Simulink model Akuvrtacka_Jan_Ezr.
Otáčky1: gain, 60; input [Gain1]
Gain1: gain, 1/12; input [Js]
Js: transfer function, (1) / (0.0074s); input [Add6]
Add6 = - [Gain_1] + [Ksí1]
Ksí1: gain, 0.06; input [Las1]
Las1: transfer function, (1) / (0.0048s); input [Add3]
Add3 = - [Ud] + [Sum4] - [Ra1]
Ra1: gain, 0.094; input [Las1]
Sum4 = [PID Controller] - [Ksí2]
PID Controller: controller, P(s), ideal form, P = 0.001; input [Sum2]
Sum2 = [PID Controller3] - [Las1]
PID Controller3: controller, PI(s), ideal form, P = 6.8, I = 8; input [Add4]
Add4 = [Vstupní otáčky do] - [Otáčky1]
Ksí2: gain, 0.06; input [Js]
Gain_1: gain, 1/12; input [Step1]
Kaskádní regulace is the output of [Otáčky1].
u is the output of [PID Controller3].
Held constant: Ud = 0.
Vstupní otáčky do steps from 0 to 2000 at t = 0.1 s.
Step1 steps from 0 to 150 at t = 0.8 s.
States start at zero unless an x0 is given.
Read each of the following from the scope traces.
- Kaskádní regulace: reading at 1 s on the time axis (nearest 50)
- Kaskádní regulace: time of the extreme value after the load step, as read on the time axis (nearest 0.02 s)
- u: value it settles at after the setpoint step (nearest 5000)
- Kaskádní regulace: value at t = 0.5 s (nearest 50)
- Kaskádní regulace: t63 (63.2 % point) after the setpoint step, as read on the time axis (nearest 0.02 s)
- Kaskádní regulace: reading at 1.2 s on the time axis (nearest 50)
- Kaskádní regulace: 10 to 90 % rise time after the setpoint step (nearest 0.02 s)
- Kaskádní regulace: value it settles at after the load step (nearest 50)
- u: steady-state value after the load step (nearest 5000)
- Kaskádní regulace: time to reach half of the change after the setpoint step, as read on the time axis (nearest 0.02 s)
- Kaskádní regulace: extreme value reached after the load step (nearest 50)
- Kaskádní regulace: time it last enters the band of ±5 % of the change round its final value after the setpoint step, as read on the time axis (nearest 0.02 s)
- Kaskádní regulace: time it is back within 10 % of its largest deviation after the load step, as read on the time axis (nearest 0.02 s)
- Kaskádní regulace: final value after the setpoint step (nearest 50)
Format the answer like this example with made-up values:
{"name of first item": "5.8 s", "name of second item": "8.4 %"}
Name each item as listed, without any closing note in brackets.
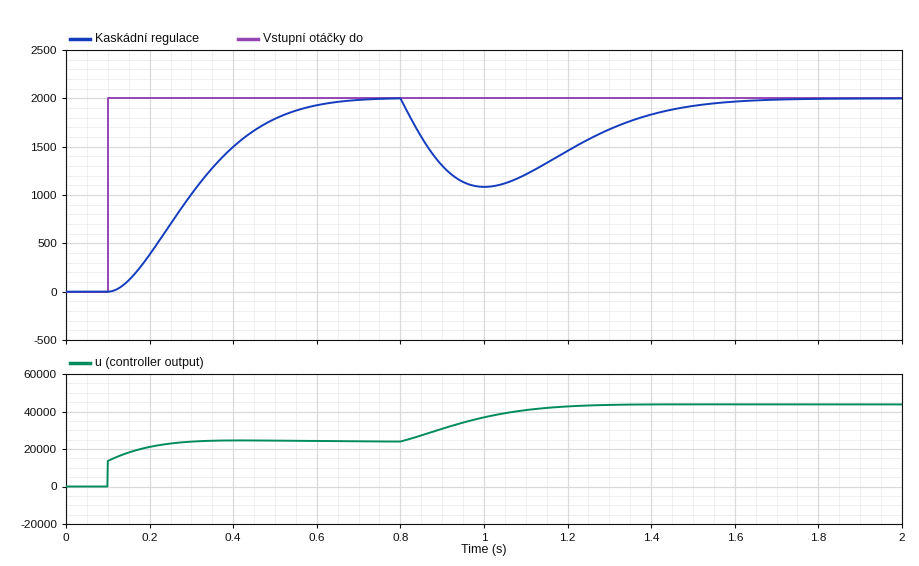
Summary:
{"Kaskádní regulace: reading at 1 s on the time axis": "1100", "Kaskádní regulace: time of the extreme value after the load step, as read on the time axis": "1.00 s", "u: value it settles at after the setpoint step": "25000", "Kaskádní regulace: value at t = 0.5 s": "1800", "Kaskádní regulace: t63 (63.2 % point) after the setpoint step, as read on the time axis": "0.34 s", "Kaskádní regulace: reading at 1.2 s on the time axis": "1450", "Kaskádní regulace: 10 to 90 % rise time after the setpoint step": "0.34 s", "Kaskádní regulace: value it settles at after the load step": "2000", "u: steady-state value after the load step": "45000", "Kaskádní regulace: time to reach half of the change after the setpoint step, as read on the time axis": "0.30 s", "Kaskádní regulace: extreme value reached after the load step": "1100", "Kaskádní regulace: time it last enters the band of ±5 % of the change round its final value after the setpoint step, as read on the time axis": "0.58 s", "Kaskádní regulace: time it is back within 10 % of its largest deviation after the load step, as read on the time axis": "1.48 s", "Kaskádní regulace: final value after the setpoint step": "2000"}
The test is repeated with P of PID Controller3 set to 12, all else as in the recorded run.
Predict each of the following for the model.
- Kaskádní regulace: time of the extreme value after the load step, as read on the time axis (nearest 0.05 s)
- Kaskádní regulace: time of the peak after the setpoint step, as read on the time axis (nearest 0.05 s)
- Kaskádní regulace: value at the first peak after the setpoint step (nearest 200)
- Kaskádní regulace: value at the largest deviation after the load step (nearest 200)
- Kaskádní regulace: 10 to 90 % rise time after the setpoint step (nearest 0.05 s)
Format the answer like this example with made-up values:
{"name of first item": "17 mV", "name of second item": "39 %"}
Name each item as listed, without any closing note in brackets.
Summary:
{"Kaskádní regulace: time of the extreme value after the load step, as read on the time axis": "0.95 s", "Kaskádní regulace: time of the peak after the setpoint step, as read on the time axis": "0.50 s", "Kaskádní regulace: value at the first peak after the setpoint step": "2200", "Kaskádní regulace: value at the largest deviation after the load step": "1200", "Kaskádní regulace: 10 to 90 % rise time after the setpoint step": "0.20 s"}
